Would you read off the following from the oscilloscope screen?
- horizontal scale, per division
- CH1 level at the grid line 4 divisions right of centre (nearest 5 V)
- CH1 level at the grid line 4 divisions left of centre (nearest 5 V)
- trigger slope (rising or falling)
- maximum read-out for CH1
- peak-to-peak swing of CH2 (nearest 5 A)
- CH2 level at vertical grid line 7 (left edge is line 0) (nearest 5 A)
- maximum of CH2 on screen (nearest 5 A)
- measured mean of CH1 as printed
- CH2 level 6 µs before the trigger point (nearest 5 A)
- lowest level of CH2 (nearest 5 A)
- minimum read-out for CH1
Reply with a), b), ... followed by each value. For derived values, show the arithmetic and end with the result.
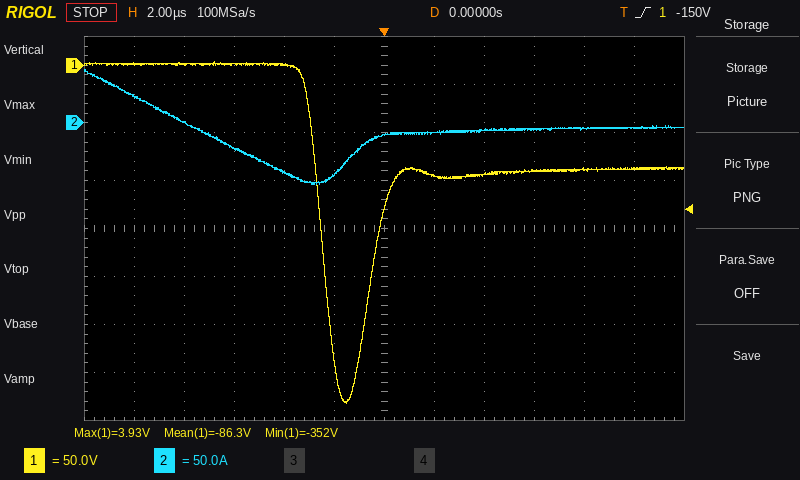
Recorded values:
a) 2 µs
b) -110 V
c) 0 V
d) rising
e) 3.93 V
f) 55 A − (-65 A) = 120 A
g) -10 A
h) 55 A
i) -86.3 V
j) -25 A
k) -65 A
l) -352 V
